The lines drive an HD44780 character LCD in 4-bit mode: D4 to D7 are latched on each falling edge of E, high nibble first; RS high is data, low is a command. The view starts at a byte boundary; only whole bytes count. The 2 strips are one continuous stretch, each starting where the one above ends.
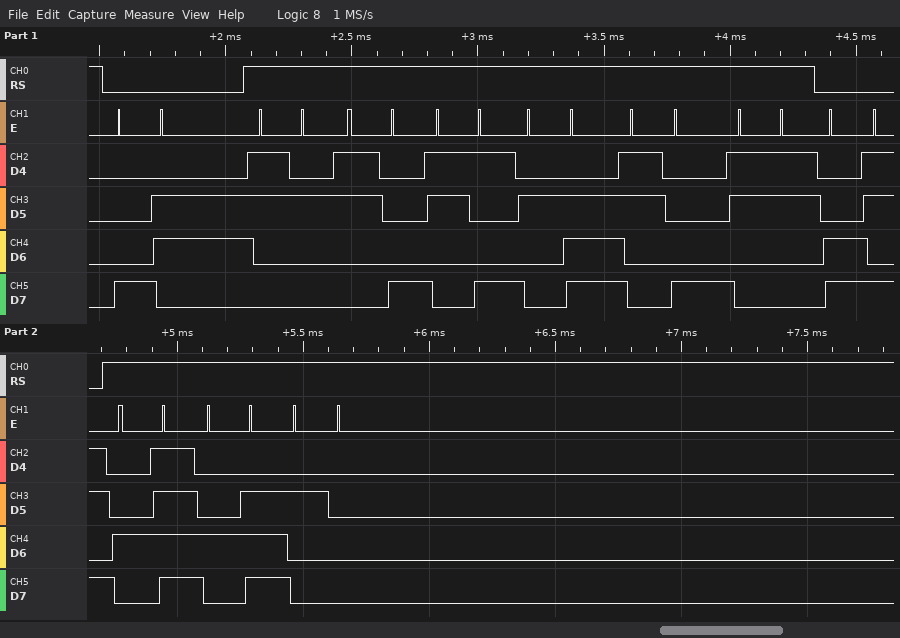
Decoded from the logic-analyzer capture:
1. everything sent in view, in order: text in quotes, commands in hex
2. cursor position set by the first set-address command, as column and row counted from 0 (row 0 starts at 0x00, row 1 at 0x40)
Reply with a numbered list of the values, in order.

1. 0x86 "289.83" 0xCB "ON "
2. column 6, row 0
